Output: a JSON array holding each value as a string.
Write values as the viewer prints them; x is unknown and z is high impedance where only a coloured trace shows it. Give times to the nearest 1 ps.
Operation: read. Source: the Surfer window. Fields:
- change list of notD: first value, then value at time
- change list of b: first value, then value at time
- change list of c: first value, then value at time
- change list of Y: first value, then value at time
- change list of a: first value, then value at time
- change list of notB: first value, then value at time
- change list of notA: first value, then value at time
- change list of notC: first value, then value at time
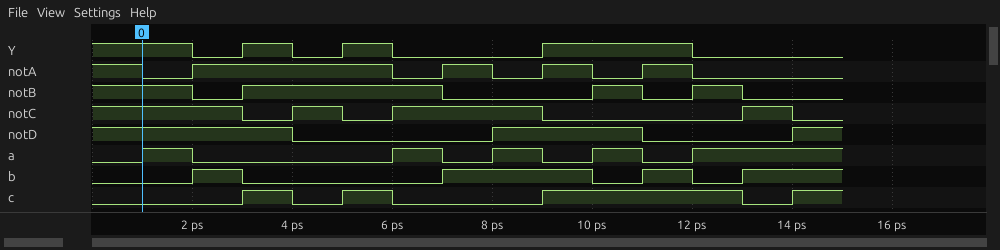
["1, 0 at 4 ps, 1 at 8 ps, 0 at 11 ps, 1 at 14 ps", "0, 1 at 2 ps, 0 at 3 ps, 1 at 7 ps, 0 at 10 ps, 1 at 11 ps, 0 at 12 ps, 1 at 13 ps", "0, 1 at 3 ps, 0 at 4 ps, 1 at 5 ps, 0 at 6 ps, 1 at 9 ps, 0 at 13 ps, 1 at 14 ps", "1, 0 at 2 ps, 1 at 3 ps, 0 at 4 ps, 1 at 5 ps, 0 at 6 ps, 1 at 9 ps, 0 at 12 ps", "0, 1 at 1 ps, 0 at 2 ps, 1 at 6 ps, 0 at 7 ps, 1 at 8 ps, 0 at 9 ps, 1 at 10 ps, 0 at 11 ps, 1 at 12 ps", "1, 0 at 2 ps, 1 at 3 ps, 0 at 7 ps, 1 at 10 ps, 0 at 11 ps, 1 at 12 ps, 0 at 13 ps", "1, 0 at 1 ps, 1 at 2 ps, 0 at 6 ps, 1 at 7 ps, 0 at 8 ps, 1 at 9 ps, 0 at 10 ps, 1 at 11 ps, 0 at 12 ps", "1, 0 at 3 ps, 1 at 4 ps, 0 at 5 ps, 1 at 6 ps, 0 at 9 ps, 1 at 13 ps, 0 at 14 ps"]
